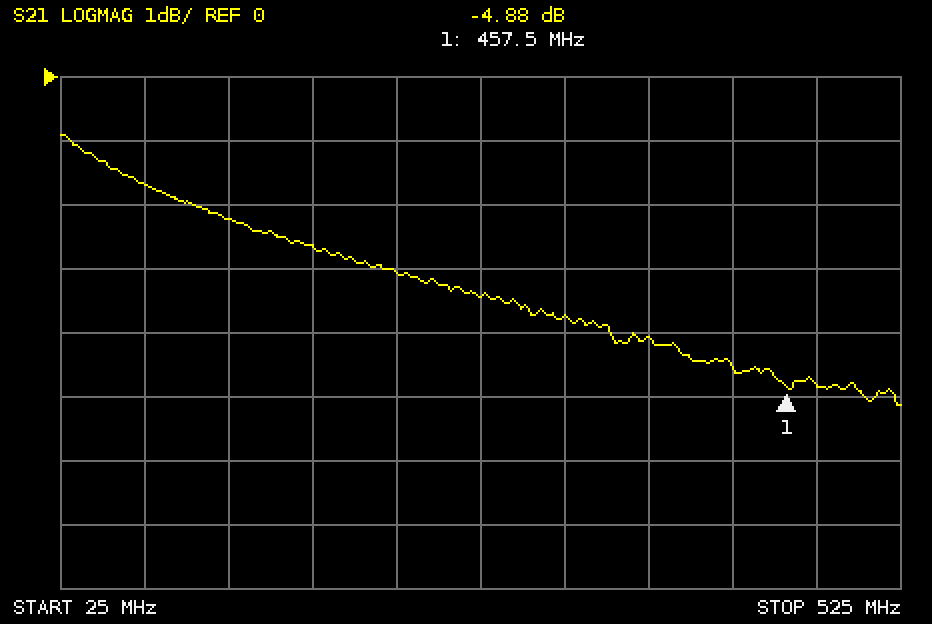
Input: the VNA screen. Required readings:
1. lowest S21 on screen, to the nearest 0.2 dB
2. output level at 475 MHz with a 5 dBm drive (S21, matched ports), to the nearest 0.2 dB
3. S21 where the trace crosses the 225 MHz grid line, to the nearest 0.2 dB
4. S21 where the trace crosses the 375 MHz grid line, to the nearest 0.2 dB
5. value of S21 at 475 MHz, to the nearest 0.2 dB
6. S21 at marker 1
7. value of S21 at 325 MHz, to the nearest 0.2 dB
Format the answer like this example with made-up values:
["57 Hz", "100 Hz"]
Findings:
["-5.2 dB", "0.2 dBm", "-3.0 dB", "-4.0 dB", "-4.8 dB", "-4.88 dB", "-3.8 dB"]
